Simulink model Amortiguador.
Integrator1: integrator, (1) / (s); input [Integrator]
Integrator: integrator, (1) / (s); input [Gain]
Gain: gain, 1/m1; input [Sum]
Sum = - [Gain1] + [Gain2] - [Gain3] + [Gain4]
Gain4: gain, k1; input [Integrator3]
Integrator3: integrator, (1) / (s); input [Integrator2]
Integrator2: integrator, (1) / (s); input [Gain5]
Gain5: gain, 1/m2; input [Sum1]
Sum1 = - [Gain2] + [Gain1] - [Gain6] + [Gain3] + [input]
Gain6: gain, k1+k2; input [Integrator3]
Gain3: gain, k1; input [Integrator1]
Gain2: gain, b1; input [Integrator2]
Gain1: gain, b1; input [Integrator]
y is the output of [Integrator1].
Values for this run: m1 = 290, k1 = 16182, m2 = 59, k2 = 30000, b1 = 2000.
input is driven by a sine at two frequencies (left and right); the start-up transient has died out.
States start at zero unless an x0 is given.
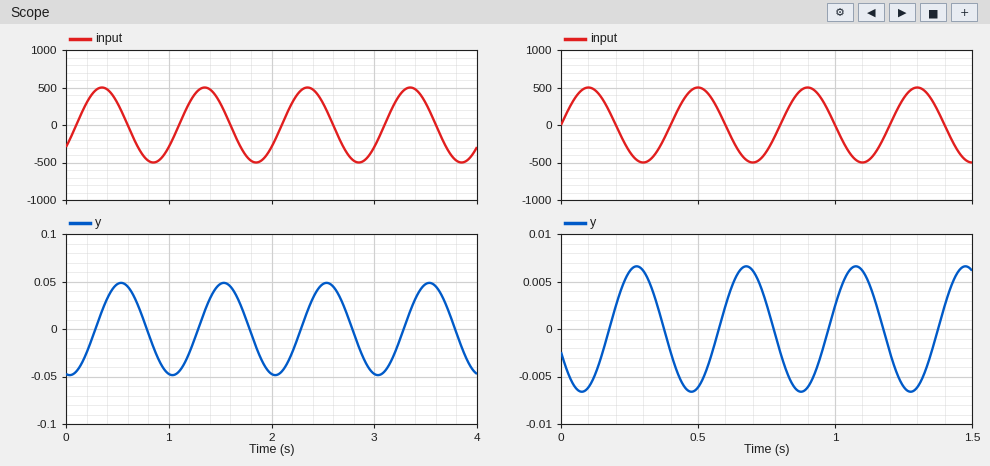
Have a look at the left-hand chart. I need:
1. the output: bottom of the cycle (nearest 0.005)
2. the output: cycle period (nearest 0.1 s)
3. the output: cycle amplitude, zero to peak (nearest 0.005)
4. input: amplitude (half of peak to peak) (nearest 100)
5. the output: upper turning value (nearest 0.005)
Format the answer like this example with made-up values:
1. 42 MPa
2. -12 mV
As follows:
1. -0.050
2. 1.0 s
3. 0.050
4. 500
5. 0.050
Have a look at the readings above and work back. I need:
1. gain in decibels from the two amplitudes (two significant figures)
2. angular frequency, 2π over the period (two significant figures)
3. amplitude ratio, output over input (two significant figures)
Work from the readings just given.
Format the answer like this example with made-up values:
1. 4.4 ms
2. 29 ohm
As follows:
1. -80 dB
2. 6.3 rad/s
3. 0.00010
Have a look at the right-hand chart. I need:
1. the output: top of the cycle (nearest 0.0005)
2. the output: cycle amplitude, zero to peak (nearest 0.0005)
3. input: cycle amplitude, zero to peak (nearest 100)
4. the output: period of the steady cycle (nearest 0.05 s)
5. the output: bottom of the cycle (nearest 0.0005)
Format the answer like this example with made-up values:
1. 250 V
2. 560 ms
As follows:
1. 0.0065
2. 0.0065
3. 500
4. 0.40 s
5. -0.0065
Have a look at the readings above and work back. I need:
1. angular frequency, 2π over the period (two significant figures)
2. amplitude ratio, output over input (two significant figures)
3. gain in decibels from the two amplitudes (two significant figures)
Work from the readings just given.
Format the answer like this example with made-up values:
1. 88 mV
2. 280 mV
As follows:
1. 16 rad/s
2. 0.000013
3. -98 dB
